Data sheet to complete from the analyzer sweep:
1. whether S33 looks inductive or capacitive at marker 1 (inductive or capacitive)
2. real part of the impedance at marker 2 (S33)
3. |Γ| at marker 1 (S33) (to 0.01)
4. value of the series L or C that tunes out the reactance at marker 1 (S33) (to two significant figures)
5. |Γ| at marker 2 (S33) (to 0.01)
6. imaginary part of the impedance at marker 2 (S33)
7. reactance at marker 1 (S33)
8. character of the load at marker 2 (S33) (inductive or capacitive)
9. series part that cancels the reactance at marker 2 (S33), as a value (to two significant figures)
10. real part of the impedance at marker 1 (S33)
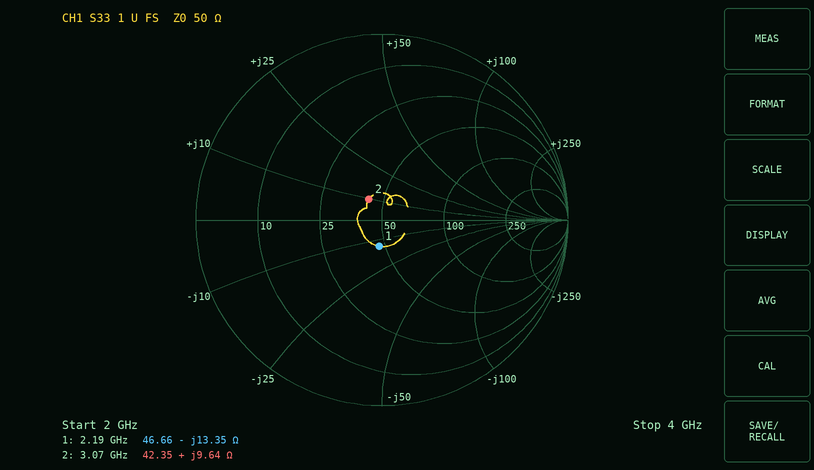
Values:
capacitive
42.35 Ω
0.14
970 pH
0.13
+9.64 Ω
-13.35 Ω
inductive
5.4 pF
46.66 Ω
